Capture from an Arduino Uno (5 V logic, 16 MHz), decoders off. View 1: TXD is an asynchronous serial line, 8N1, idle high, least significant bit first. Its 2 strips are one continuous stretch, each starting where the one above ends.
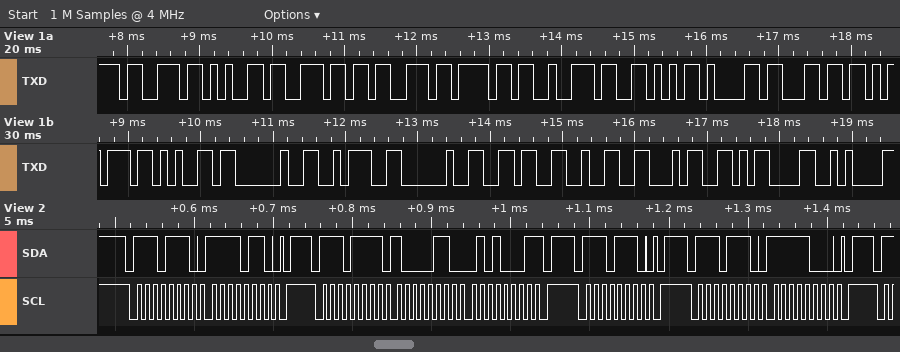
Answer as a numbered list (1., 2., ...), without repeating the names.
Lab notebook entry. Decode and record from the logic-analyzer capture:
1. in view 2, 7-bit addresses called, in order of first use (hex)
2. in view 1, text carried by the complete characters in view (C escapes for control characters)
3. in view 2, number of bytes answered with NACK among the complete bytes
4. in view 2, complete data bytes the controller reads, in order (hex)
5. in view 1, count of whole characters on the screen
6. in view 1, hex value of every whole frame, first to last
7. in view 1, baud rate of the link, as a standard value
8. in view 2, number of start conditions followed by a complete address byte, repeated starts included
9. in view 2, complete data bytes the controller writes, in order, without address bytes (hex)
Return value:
1. 0x77
2. "sensorValue : 624\r\n"
3. 1
4. 86 51
5. 19
6. 0x73 0x65 0x6E 0x73 0x6F 0x72 0x56 0x61 0x6C 0x75 0x65 0x20 0x3A 0x20 0x36 0x32 0x34 0x0D 0x0A
7. 9600 baud
8. 4
9. F6 F8
